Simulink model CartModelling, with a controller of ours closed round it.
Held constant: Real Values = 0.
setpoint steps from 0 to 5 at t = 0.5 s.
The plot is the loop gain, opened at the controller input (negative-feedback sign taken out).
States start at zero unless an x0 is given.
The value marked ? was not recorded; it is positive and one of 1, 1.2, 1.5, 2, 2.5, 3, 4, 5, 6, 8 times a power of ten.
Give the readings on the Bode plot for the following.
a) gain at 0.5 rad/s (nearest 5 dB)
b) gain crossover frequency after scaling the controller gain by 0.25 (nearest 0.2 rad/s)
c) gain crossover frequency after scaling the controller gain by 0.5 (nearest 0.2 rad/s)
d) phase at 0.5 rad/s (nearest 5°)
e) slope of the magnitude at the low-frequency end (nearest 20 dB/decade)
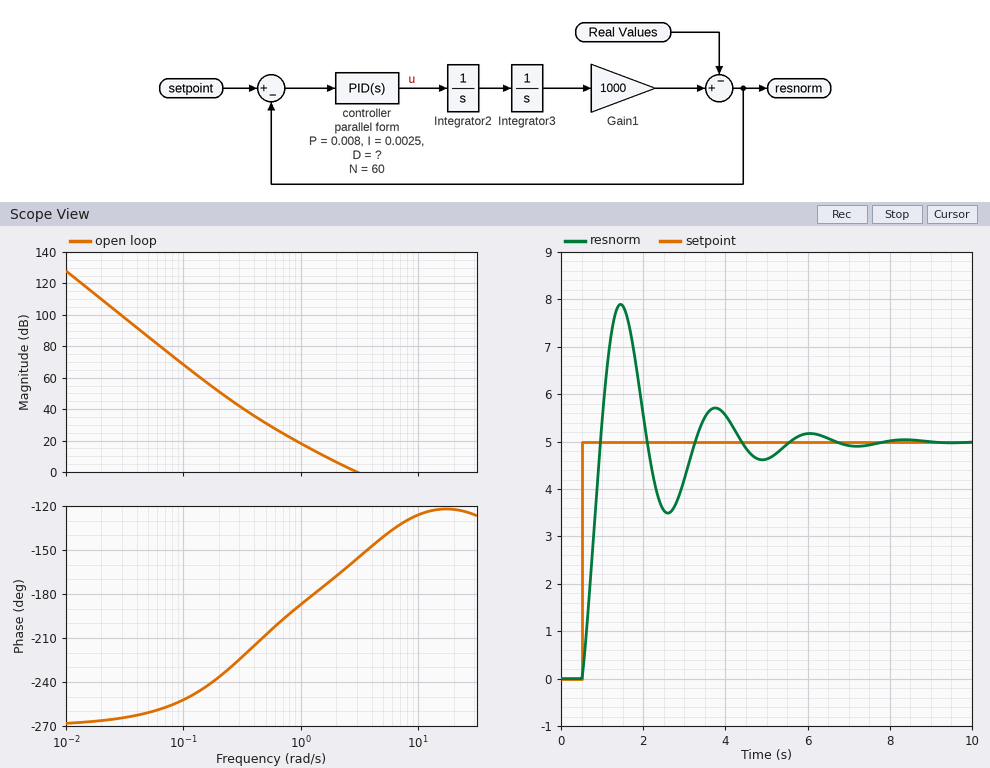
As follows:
30 dB
1.4 rad/s
2.0 rad/s
-210°
-60 dB/decade
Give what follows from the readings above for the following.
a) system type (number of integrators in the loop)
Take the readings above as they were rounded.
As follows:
3
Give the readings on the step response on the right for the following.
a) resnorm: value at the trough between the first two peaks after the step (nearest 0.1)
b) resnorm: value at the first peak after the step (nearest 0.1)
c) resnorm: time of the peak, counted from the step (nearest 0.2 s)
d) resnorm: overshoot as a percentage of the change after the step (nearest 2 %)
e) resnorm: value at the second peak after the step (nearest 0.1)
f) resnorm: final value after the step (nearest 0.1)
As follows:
3.5
7.9
1.0 s
58 %
5.7
5.0
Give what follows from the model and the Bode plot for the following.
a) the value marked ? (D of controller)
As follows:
0.0015
